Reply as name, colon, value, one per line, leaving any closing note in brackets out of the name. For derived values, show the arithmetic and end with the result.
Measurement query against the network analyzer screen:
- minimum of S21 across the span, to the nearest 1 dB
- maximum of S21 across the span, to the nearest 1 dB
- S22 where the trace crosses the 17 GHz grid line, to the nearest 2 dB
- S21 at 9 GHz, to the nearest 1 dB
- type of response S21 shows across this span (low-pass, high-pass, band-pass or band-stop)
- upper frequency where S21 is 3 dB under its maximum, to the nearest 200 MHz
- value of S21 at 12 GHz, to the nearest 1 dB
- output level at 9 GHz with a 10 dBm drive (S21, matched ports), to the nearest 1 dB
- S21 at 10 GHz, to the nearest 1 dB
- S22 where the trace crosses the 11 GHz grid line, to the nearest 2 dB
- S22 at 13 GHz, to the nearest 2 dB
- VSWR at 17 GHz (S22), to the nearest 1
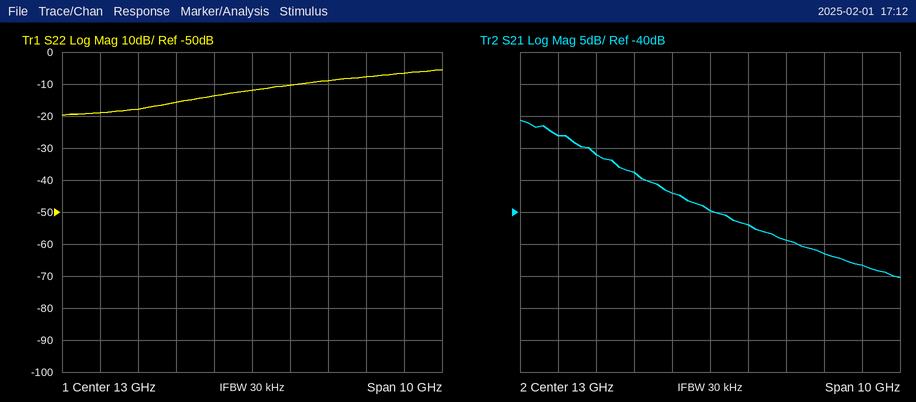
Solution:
minimum of S21 across the span, to the nearest 1 dB: -50 dB
maximum of S21 across the span, to the nearest 1 dB: -26 dB
S22 where the trace crosses the 17 GHz grid line, to the nearest 2 dB: -6 dB
S21 at 9 GHz, to the nearest 1 dB: -28 dB
type of response S21 shows across this span: low-pass
upper frequency where S21 is 3 dB under its maximum, to the nearest 200 MHz: 9.4 GHz
value of S21 at 12 GHz, to the nearest 1 dB: -37 dB
output level at 9 GHz with a 10 dBm drive (S21, matched ports), to the nearest 1 dB: 10 dBm + (-28 dB) = -18 dBm
S21 at 10 GHz, to the nearest 1 dB: -31 dB
S22 where the trace crosses the 11 GHz grid line, to the nearest 2 dB: -16 dB
S22 at 13 GHz, to the nearest 2 dB: -12 dB
VSWR at 17 GHz (S22), to the nearest 1: |Γ| = 10^(-6/20) = 0.5012; VSWR = (1 + 0.5012)/(1 − 0.5012) ≈ 3
